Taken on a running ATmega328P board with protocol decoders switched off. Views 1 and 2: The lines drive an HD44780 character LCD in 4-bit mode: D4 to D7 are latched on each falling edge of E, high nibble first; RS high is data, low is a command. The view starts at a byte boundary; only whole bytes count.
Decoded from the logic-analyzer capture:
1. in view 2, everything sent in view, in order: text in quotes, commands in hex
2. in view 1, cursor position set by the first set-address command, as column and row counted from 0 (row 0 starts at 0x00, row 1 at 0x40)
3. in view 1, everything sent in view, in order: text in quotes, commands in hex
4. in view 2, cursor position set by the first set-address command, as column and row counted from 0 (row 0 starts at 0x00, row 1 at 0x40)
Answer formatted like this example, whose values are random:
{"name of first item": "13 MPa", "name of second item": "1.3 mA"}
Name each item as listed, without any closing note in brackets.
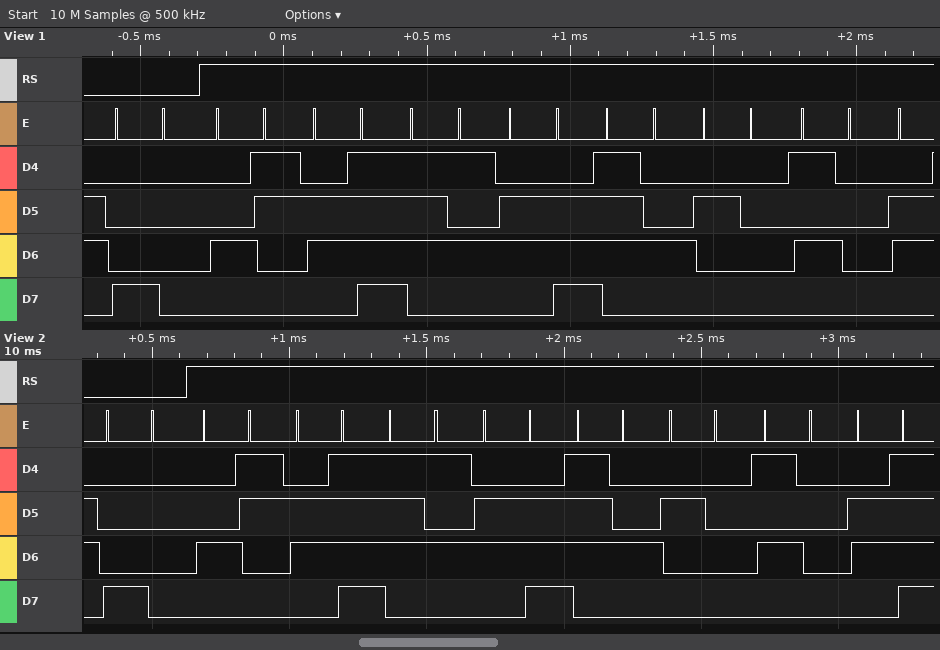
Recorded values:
{"in view 2, everything sent in view, in order: text in quotes, commands in hex": "0x80 \"Count Po\"", "in view 1, cursor position set by the first set-address command, as column and row counted from 0": "column 0, row 0", "in view 1, everything sent in view, in order: text in quotes, commands in hex": "0x80 \"Count P\"", "in view 2, cursor position set by the first set-address command, as column and row counted from 0": "column 0, row 0"}
